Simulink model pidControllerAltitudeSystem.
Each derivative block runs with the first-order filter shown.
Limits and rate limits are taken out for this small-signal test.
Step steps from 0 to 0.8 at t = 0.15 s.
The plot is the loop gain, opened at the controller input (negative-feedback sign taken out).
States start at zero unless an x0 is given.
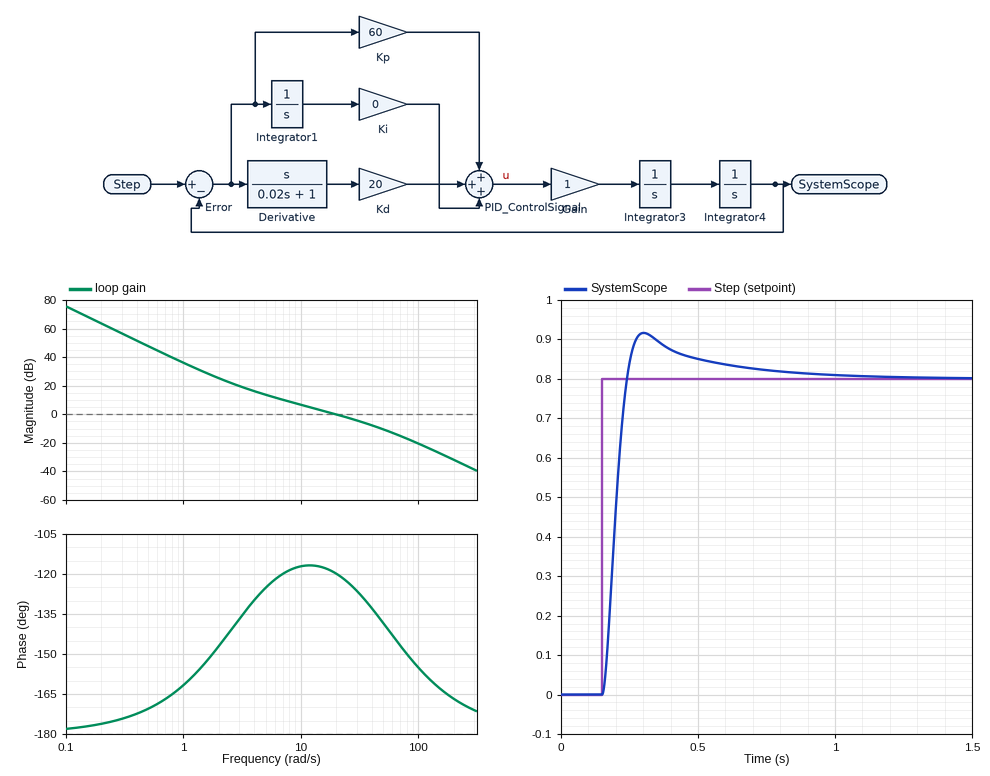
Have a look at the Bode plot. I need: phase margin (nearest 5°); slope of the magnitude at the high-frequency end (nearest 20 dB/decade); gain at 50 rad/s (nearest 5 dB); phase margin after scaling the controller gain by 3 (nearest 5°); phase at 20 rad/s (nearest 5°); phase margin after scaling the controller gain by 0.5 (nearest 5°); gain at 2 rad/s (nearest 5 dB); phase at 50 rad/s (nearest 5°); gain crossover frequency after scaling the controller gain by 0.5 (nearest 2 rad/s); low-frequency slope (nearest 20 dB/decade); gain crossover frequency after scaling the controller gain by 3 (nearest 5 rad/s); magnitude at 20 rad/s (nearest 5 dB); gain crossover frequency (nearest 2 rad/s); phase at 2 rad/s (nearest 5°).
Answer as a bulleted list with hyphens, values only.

- 60°
- -40 dB/decade
- -10 dB
- 45°
- -120°
- 65°
- 25 dB
- -140°
- 10 rad/s
- -40 dB/decade
- 45 rad/s
- 0 dB
- 20 rad/s
- -145°
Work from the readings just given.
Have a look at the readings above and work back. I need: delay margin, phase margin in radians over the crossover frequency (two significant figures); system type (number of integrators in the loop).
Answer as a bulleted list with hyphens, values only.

- 0.052 s
- 2
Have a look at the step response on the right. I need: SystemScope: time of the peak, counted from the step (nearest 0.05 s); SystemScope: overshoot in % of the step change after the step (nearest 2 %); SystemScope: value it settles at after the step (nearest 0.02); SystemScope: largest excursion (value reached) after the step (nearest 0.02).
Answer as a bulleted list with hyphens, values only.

- 0.15 s
- 14 %
- 0.80
- 0.92
